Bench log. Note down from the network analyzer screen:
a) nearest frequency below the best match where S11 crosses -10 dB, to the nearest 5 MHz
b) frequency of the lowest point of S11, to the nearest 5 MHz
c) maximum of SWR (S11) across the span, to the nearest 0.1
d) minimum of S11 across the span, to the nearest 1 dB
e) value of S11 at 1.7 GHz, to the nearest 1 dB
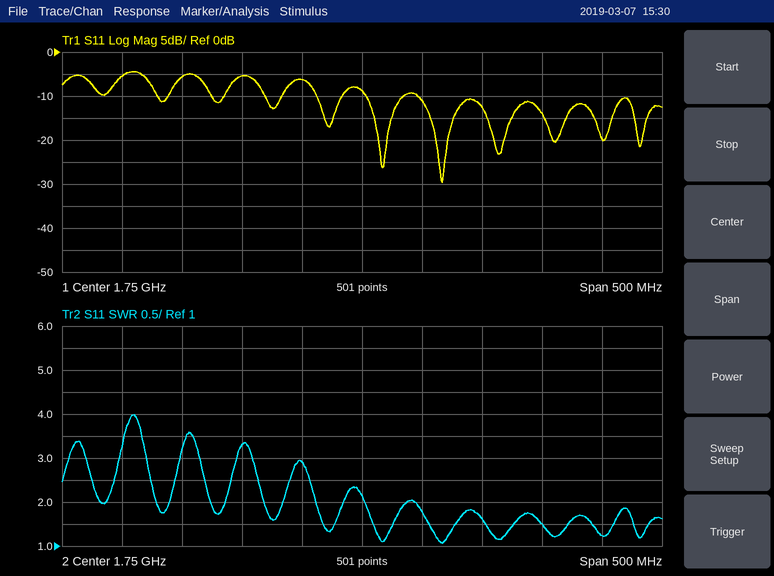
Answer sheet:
1.795 GHz
1.815 GHz
4.0
-30 dB
-6 dB
